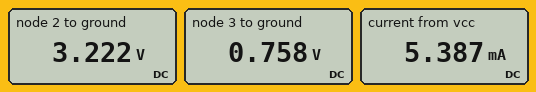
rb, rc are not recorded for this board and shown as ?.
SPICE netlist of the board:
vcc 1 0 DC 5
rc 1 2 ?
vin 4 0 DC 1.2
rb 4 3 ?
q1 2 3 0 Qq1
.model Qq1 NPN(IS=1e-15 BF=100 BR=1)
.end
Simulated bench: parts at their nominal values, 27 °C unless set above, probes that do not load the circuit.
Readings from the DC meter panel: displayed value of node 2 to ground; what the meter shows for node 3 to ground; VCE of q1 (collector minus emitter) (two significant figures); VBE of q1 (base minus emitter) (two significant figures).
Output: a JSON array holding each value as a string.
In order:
["3.222 V", "0.758 V", "3.2 V", "760 mV"]
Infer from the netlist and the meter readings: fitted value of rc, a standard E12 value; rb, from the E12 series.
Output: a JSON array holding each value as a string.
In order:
["330 Ω", "8.2 kΩ"]
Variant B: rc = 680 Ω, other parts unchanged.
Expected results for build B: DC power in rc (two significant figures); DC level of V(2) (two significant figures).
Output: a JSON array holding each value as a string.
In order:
["20 mW", "1.3 V"]
